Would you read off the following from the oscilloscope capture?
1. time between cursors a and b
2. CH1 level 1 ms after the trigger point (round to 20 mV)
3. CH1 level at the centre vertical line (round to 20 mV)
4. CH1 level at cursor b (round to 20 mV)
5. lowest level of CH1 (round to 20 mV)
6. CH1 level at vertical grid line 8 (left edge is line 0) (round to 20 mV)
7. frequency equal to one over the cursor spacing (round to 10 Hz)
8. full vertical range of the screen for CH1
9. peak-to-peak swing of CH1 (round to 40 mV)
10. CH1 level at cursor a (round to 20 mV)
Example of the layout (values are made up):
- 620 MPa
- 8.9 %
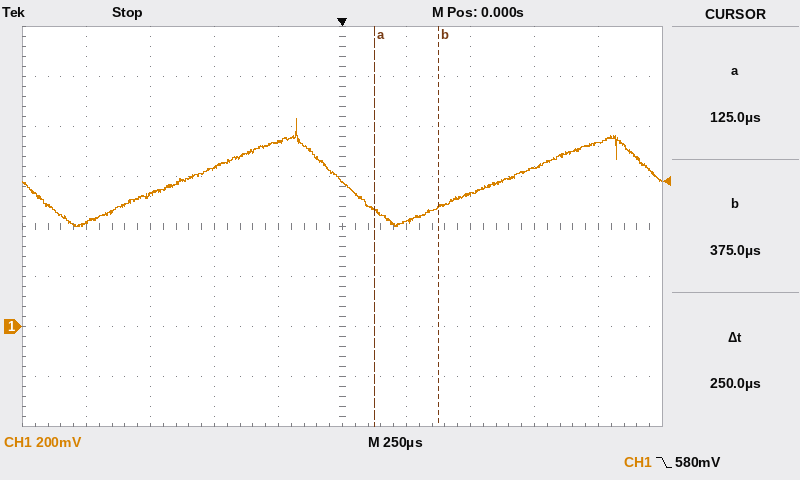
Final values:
- 250 µs
- 740 mV
- 580 mV
- 480 mV
- 400 mV
- 640 mV
- 4.00 kHz
- 1.6 V
- 440 mV
- 460 mV
